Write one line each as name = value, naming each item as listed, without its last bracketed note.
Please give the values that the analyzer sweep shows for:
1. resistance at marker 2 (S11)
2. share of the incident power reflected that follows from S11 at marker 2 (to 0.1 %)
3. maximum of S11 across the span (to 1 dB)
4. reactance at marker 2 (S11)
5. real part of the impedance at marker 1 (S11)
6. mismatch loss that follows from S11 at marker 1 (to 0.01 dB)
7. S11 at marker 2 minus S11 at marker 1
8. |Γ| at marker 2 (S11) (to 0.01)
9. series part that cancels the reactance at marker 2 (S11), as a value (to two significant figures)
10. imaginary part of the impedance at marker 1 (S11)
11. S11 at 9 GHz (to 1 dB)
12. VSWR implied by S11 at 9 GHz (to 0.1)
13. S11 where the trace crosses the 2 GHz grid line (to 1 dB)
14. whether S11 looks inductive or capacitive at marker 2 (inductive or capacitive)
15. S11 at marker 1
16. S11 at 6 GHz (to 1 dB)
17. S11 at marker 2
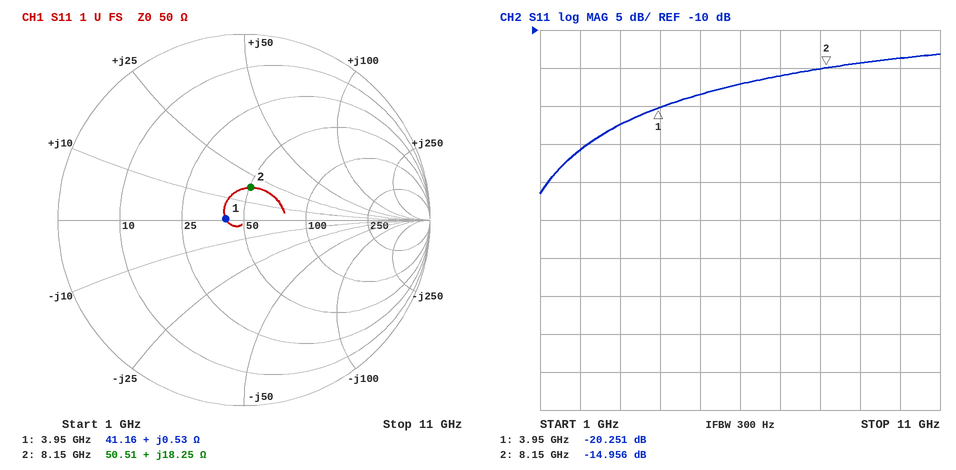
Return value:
resistance at marker 2 = 50.51 Ω
share of the incident power reflected that follows from S11 at marker 2 = 3.2 %
maximum of S11 across the span = -13 dB
reactance at marker 2 = +18.25 Ω
real part of the impedance at marker 1 = 41.16 Ω
mismatch loss that follows from S11 at marker 1 = 0.04 dB
S11 at marker 2 minus S11 at marker 1 = 5.295 dB
|Γ| at marker 2 (S11) = 0.18
series part that cancels the reactance at marker 2 (S11), as a value = 1.1 pF
imaginary part of the impedance at marker 1 = +0.53 Ω
S11 at 9 GHz = -14 dB
VSWR implied by S11 at 9 GHz = 1.5
S11 where the trace crosses the 2 GHz grid line = -26 dB
whether S11 looks inductive or capacitive at marker 2 = inductive
S11 at marker 1 = -20.251 dB
S11 at 6 GHz = -17 dB
S11 at marker 2 = -14.956 dB
